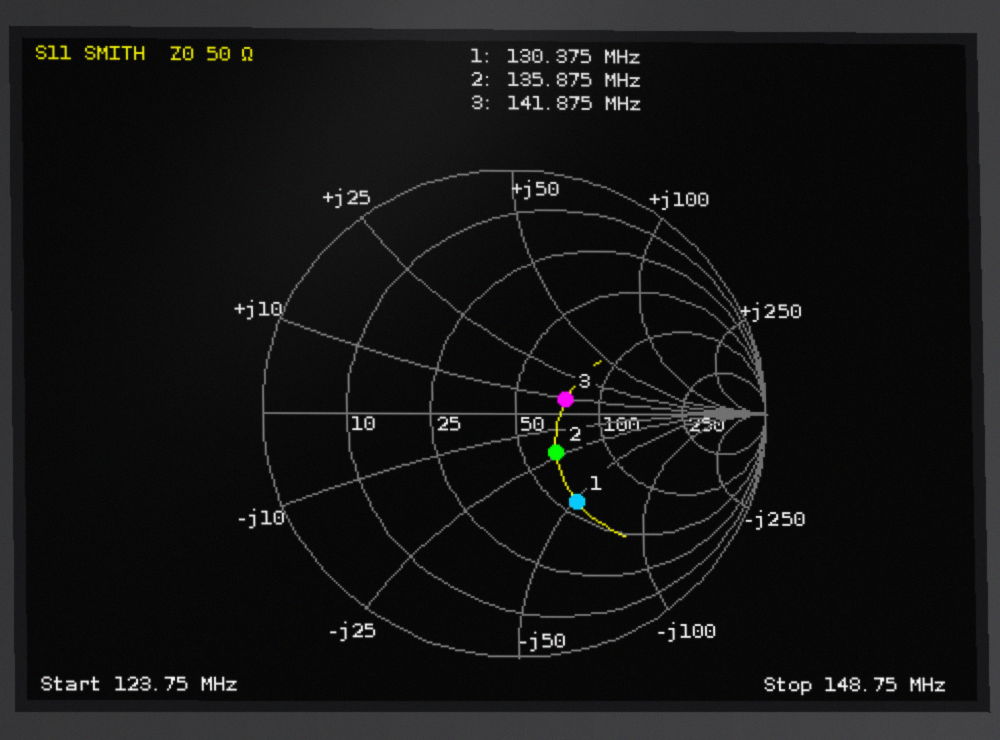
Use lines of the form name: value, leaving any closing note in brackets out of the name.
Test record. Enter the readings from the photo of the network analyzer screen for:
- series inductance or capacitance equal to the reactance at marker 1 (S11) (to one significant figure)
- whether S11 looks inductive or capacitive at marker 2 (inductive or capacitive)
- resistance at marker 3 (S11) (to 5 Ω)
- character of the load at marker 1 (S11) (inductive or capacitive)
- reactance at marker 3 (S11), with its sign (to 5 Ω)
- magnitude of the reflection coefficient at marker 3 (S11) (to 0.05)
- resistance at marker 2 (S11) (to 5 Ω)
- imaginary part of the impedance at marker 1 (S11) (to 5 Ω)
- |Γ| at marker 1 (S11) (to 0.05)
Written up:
series inductance or capacitance equal to the reactance at marker 1 (S11): 20 pF
whether S11 looks inductive or capacitive at marker 2: capacitive
resistance at marker 3 (S11): 75 Ω
character of the load at marker 1 (S11): capacitive
reactance at marker 3 (S11), with its sign: +10 Ω
magnitude of the reflection coefficient at marker 3 (S11): 0.20
resistance at marker 2 (S11): 65 Ω
imaginary part of the impedance at marker 1 (S11): -50 Ω
|Γ| at marker 1 (S11): 0.45
